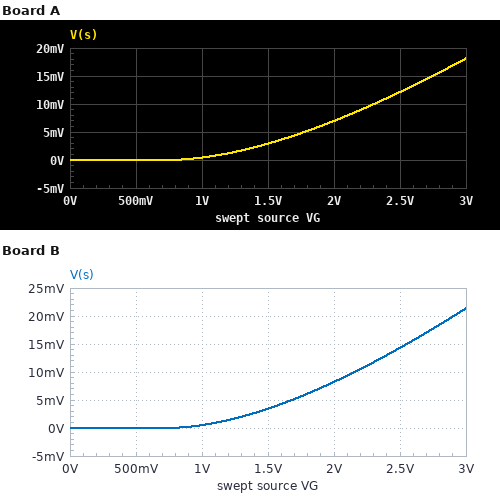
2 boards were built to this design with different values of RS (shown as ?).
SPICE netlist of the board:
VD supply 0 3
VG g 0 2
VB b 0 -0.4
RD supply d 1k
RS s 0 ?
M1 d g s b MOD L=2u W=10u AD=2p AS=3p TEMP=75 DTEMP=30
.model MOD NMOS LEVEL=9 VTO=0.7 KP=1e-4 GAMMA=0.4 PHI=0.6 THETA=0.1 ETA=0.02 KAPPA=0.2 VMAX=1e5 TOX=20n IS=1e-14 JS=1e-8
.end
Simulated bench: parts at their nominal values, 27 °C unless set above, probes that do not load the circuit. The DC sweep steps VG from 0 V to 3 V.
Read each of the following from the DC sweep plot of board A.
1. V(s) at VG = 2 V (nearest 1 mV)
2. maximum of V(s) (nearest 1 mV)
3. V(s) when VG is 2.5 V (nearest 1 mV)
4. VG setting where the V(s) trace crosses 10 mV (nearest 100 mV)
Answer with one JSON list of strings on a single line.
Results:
["7 mV", "18 mV", "12 mV", "2.3 V"]
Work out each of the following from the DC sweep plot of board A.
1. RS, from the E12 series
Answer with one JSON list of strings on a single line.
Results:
["33 Ω"]
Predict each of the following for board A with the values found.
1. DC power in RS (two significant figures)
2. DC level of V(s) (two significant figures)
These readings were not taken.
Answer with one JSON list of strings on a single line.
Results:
["1.5 µW", "7.0 mV"]
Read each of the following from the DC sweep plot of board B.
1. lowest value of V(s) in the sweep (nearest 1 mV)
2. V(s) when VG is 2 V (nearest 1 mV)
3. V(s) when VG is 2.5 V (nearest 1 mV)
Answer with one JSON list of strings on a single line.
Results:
["0 V", "8 mV", "14 mV"]
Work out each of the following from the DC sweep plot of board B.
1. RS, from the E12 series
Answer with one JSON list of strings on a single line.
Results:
["39 Ω"]
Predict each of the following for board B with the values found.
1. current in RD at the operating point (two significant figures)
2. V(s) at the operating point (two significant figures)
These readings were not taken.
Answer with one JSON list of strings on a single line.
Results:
["210 µA", "8.2 mV"]
